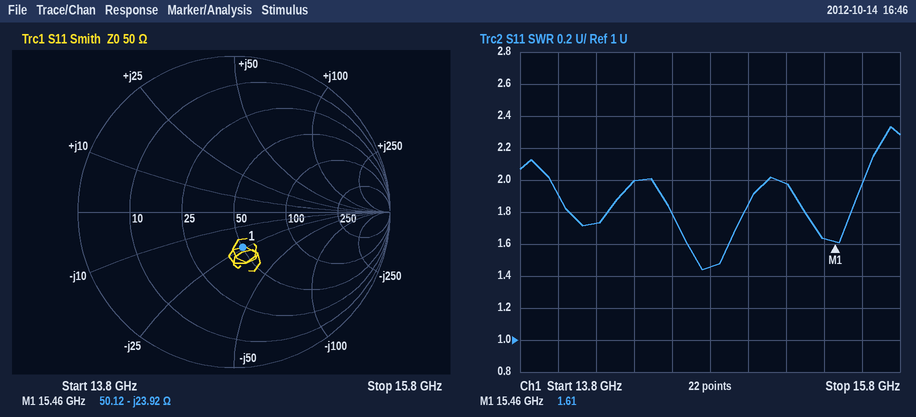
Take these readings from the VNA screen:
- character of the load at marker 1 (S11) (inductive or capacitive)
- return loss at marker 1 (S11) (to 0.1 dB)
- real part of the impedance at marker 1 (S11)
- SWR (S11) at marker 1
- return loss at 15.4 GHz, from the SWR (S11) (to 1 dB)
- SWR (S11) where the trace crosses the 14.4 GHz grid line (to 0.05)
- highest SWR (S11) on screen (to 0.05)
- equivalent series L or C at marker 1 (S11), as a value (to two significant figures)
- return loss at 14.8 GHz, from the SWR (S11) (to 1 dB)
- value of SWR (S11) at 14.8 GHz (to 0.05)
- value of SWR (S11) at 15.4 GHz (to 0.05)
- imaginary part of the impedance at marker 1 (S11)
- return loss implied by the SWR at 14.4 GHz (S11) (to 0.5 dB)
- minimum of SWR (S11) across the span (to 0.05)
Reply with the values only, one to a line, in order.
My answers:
capacitive
12.7 dB
50.12 Ω
1.61
12 dB
2.00
2.35
430 fF
15 dB
1.45
1.65
-23.92 Ω
9.5 dB
1.45
